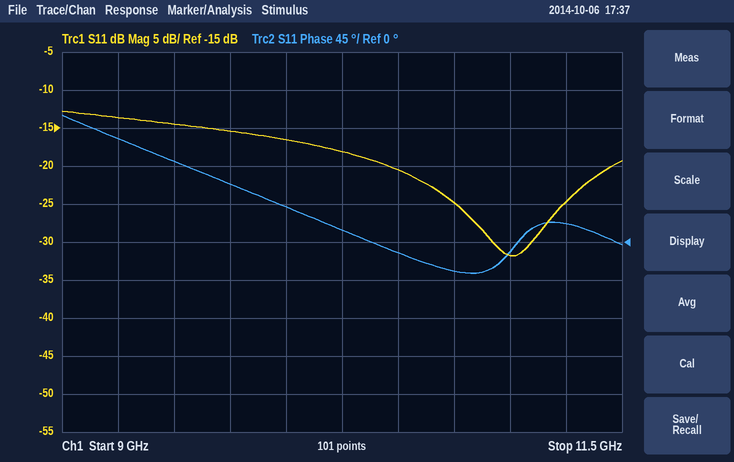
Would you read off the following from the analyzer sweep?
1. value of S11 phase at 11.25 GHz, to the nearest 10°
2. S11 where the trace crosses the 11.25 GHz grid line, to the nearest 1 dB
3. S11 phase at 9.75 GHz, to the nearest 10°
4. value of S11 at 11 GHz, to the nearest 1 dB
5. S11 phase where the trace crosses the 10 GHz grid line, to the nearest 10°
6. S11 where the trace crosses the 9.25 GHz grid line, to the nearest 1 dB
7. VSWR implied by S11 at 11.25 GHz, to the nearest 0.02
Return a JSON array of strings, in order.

["20°", "-25 dB", "70°", "-32 dB", "40°", "-14 dB", "1.12"]
